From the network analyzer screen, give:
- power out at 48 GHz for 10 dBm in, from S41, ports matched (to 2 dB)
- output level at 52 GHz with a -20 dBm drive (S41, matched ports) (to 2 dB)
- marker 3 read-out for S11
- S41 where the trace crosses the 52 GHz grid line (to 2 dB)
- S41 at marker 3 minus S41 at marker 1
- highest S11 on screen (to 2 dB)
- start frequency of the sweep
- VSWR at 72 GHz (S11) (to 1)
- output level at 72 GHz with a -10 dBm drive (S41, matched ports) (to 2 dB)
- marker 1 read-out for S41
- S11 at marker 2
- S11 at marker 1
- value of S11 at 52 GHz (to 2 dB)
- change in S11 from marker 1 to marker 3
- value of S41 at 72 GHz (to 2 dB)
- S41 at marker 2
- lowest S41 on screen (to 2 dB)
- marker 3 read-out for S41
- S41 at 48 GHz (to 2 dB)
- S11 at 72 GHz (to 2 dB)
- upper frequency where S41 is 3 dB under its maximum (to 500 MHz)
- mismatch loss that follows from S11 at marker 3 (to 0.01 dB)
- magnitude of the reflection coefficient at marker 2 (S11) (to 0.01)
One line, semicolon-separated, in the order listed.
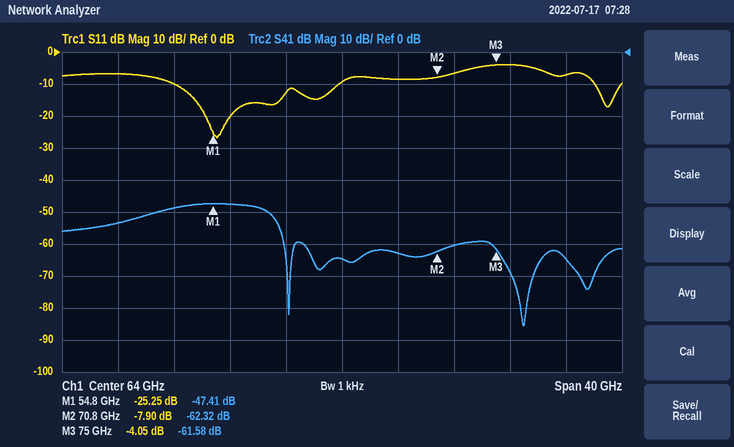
-44 dBm; -68 dBm; -4.05 dB; -48 dB; -14.17 dB; -4 dB; 44 GHz; 3; -70 dBm; -47.41 dB; -7.90 dB; -25.25 dB; -10 dB; 21.20 dB; -60 dB; -62.32 dB; -86 dB; -61.58 dB; -54 dB; -6 dB; 59.0 GHz; 2.17 dB; 0.40
